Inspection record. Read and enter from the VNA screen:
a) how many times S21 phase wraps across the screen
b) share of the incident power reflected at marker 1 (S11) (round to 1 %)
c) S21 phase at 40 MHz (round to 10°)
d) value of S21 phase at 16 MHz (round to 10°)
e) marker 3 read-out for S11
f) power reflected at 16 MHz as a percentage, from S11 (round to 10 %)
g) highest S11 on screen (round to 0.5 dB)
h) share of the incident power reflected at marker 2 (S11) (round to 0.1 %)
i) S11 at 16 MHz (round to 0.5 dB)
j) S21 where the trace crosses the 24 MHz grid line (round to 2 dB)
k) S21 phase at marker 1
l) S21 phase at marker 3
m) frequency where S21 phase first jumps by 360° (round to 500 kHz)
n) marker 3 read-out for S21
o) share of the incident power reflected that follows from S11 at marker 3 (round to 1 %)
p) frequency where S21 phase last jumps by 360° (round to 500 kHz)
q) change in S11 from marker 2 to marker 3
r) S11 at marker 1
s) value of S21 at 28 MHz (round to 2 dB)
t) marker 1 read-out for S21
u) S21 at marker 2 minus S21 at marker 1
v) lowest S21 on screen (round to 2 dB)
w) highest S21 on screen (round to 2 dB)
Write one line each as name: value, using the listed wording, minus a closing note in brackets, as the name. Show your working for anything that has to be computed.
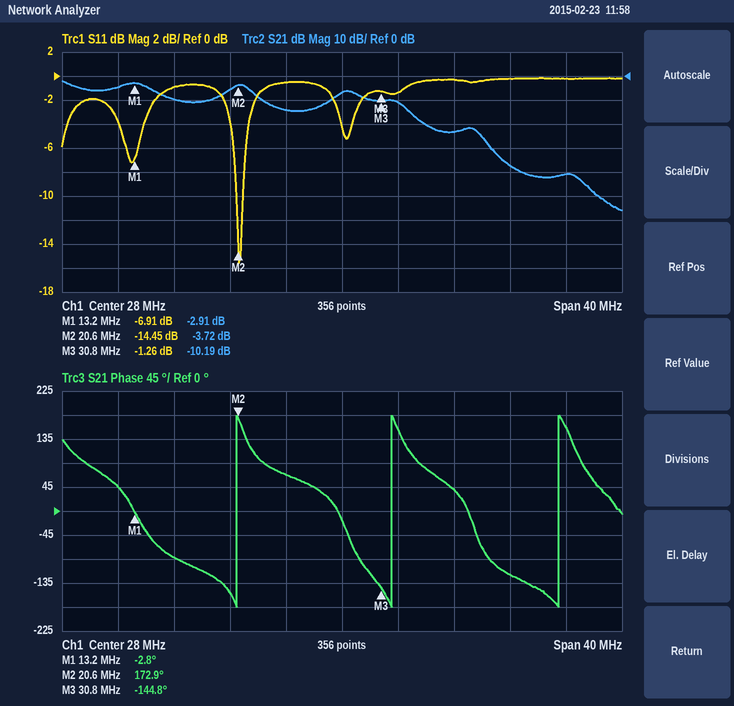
how many times S21 phase wraps across the screen: 3
share of the incident power reflected at marker 1 (S11): 10^(-6.91/10) ≈ 20 %
S21 phase at 40 MHz: -120°
value of S21 phase at 16 MHz: -90°
marker 3 read-out for S11: -1.26 dB
power reflected at 16 MHz as a percentage, from S11: 10^(-1/10) ≈ 79.4 %, so 80 % to the nearest 10 %
highest S11 on screen: 0.0 dB
share of the incident power reflected at marker 2 (S11): 10^(-14.45/10) ≈ 3.6 %
S11 at 16 MHz: -1.0 dB
S21 where the trace crosses the 24 MHz grid line: -14 dB
S21 phase at marker 1: -2.8°
S21 phase at marker 3: -144.8°
frequency where S21 phase first jumps by 360°: 20.5 MHz
marker 3 read-out for S21: -10.19 dB
share of the incident power reflected that follows from S11 at marker 3: 10^(-1.26/10) ≈ 75 %
frequency where S21 phase last jumps by 360°: 43.5 MHz
change in S11 from marker 2 to marker 3: -1.26 − (-14.45) = 13.19 dB
S11 at marker 1: -6.91 dB
value of S21 at 28 MHz: -6 dB
marker 1 read-out for S21: -2.91 dB
S21 at marker 2 minus S21 at marker 1: -3.72 − (-2.91) = -0.81 dB
lowest S21 on screen: -56 dB
highest S21 on screen: -2 dB
